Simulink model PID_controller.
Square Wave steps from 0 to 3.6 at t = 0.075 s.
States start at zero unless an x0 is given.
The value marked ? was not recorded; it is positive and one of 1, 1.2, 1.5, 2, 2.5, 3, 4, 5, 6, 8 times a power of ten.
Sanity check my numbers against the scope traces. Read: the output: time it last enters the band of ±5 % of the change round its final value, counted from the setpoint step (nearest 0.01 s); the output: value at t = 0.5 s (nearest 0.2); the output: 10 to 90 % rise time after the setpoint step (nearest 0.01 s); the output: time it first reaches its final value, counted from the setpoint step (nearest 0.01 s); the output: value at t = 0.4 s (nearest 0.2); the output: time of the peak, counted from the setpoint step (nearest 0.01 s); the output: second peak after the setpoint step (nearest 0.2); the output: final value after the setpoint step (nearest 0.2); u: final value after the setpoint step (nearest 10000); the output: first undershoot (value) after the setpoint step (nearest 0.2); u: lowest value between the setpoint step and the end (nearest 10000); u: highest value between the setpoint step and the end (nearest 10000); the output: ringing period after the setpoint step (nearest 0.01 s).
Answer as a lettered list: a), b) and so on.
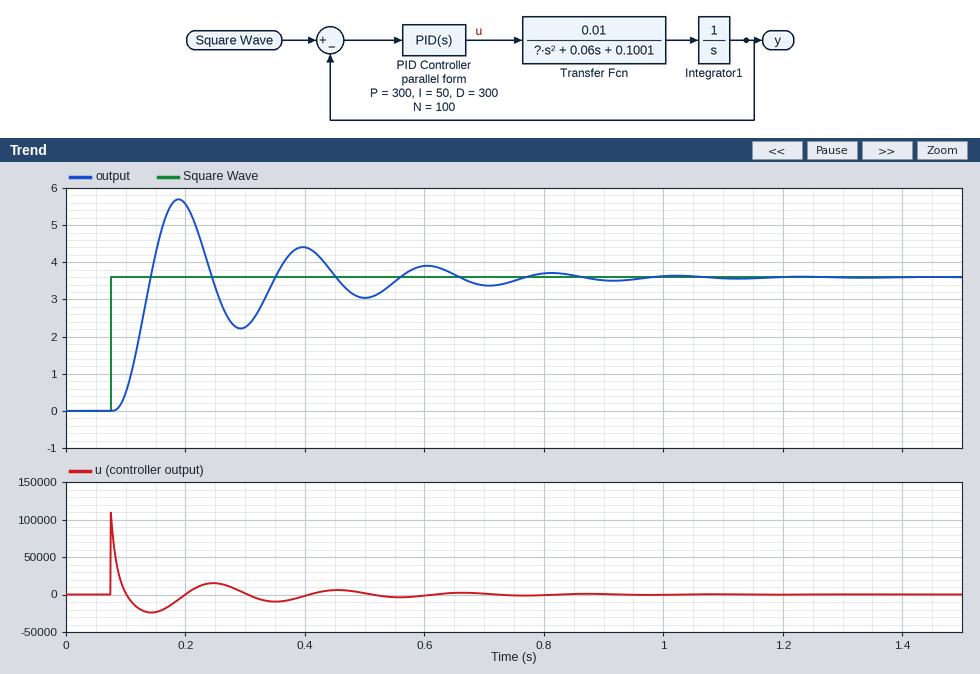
a) 0.66 s
b) 3.0
c) 0.04 s
d) 0.07 s
e) 4.4
f) 0.11 s
g) 4.4
h) 3.6
i) 0
j) 2.2
k) -20000
l) 110000
m) 0.21 s
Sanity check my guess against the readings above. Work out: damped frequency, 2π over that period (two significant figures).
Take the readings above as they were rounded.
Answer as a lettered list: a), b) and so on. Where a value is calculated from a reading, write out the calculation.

a) 2π / 0.21 = 30 rad/s
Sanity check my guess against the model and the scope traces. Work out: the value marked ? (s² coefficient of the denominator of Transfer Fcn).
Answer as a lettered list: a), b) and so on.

a) 0.003
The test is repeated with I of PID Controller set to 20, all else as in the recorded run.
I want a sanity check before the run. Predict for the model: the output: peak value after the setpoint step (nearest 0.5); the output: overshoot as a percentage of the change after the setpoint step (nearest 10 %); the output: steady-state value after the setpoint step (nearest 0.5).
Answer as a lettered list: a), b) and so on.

a) 5.5
b) 60 %
c) 3.5
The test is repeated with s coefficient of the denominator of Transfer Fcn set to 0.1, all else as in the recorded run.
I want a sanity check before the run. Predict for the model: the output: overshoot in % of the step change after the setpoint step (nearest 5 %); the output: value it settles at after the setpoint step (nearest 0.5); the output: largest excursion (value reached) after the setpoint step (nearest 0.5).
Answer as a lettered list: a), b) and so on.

a) 30 %
b) 3.5
c) 4.5
